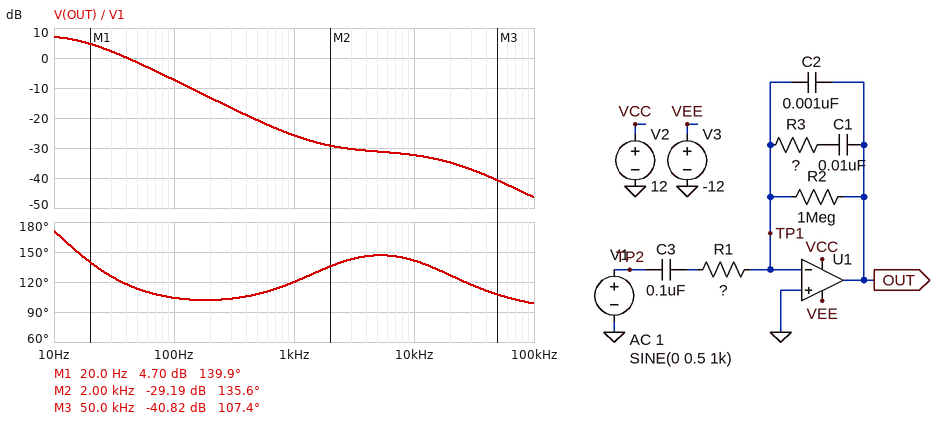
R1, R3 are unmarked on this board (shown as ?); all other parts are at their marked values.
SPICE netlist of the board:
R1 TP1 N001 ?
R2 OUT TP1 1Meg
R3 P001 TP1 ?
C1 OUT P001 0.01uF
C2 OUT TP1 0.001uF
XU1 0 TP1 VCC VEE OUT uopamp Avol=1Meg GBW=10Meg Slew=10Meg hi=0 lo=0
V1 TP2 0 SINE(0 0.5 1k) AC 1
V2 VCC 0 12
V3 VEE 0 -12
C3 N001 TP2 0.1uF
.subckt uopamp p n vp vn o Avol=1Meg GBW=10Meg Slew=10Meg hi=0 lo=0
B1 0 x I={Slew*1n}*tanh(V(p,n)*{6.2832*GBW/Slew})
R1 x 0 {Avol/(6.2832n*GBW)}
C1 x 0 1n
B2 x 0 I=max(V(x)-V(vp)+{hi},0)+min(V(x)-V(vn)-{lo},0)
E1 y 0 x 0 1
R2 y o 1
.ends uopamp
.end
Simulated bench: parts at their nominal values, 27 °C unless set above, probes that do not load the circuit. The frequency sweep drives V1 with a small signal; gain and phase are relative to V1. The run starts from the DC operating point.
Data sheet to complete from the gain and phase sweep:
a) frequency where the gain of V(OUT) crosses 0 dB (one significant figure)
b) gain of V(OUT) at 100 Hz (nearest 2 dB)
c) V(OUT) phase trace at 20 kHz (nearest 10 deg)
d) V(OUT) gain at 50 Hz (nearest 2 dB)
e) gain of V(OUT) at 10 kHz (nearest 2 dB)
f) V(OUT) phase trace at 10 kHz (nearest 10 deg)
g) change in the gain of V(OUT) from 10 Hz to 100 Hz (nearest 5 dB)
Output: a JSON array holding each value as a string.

["40 Hz", "-8 dB", "130 deg", "-2 dB", "-32 dB", "140 deg", "-15 dB"]
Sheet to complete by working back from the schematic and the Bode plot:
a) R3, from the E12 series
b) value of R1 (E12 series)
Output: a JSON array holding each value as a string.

["10 kΩ", "330 kΩ"]
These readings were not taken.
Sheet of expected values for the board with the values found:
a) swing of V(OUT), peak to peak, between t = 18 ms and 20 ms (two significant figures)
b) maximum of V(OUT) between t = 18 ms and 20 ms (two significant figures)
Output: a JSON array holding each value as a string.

["52 mV", "26 mV"]
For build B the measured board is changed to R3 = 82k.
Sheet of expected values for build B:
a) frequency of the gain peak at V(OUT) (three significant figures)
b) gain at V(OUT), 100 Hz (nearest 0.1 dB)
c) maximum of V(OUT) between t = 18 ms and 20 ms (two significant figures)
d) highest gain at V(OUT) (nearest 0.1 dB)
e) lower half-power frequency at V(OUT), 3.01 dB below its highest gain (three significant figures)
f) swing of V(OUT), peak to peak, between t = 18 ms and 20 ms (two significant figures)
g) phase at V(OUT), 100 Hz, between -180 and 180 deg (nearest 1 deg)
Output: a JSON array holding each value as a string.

["8.10 Hz", "-6.8 dB", "99 mV", "7.0 dB", "3.05 Hz", "200 mV", "125 deg"]
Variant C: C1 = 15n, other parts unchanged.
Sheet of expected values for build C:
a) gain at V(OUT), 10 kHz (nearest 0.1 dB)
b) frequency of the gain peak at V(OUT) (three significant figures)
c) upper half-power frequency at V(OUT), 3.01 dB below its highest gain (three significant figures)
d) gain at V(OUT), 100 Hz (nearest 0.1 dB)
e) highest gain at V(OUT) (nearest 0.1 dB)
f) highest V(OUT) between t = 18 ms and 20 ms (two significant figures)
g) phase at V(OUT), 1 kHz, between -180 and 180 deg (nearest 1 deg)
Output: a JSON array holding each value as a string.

["-32.2 dB", "6.90 Hz", "17.4 Hz", "-10.5 dB", "6.2 dB", "20 mV", "131 deg"]
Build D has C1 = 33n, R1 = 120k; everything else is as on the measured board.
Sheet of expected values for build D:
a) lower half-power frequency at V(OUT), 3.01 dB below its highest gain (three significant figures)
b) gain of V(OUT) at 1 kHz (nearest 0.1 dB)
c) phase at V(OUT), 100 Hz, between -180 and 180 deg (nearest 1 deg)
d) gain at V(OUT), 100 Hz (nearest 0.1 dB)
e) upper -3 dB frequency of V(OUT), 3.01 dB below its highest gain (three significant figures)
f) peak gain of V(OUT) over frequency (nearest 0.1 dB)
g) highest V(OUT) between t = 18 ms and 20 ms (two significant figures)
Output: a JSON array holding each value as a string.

["2.95 Hz", "-21.0 dB", "112 deg", "-8.2 dB", "20.9 Hz", "6.7 dB", "45 mV"]
